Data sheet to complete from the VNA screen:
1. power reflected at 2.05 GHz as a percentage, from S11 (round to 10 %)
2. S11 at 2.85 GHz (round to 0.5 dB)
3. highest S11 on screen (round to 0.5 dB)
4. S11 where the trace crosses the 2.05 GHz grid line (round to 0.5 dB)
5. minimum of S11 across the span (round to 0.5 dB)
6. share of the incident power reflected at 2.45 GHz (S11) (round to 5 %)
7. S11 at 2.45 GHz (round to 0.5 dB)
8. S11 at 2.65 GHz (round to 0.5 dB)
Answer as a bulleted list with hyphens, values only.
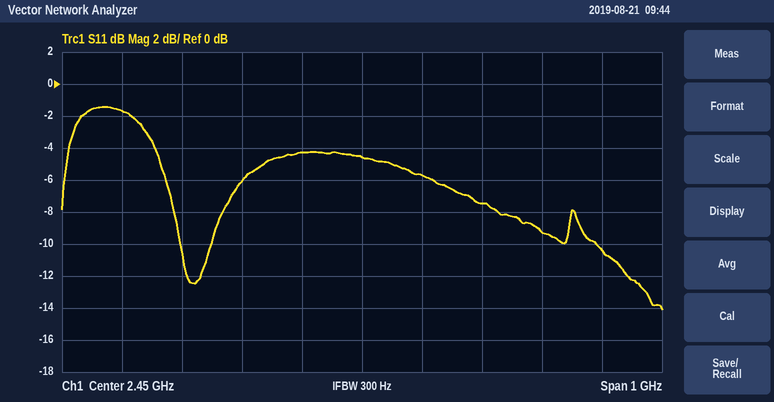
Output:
- 70 %
- -10.5 dB
- -1.5 dB
- -1.5 dB
- -14.0 dB
- 35 %
- -4.5 dB
- -7.5 dB
